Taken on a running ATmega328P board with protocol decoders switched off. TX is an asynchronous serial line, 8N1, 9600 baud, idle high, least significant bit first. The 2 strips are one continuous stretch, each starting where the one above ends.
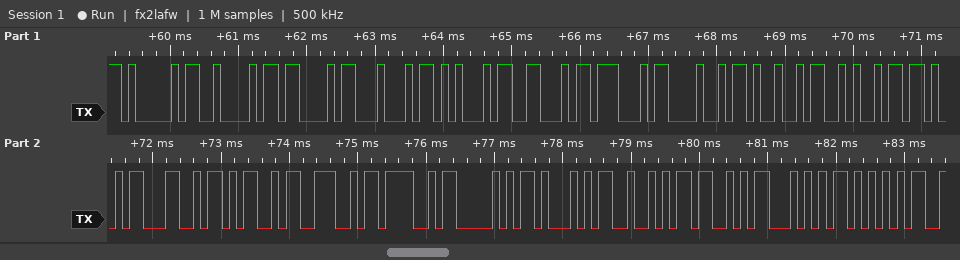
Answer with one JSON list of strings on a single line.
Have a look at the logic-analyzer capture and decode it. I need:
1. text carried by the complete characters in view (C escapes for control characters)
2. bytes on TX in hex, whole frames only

["\"ABCDEFGHIJKLMNOPQRSTU\"", "41 42 43 44 45 46 47 48 49 4A 4B 4C 4D 4E 4F 50 51 52 53 54 55"]
